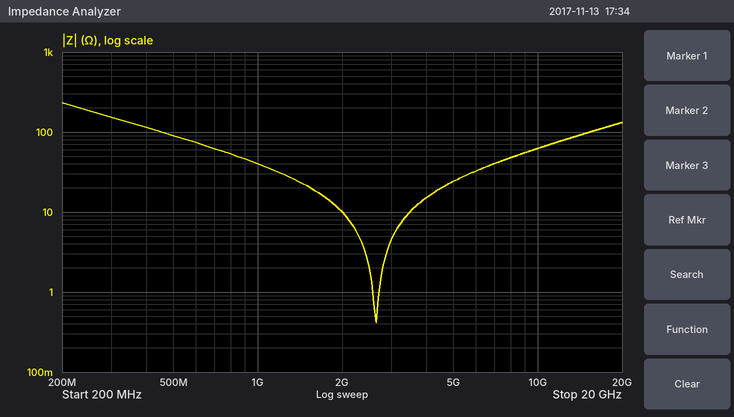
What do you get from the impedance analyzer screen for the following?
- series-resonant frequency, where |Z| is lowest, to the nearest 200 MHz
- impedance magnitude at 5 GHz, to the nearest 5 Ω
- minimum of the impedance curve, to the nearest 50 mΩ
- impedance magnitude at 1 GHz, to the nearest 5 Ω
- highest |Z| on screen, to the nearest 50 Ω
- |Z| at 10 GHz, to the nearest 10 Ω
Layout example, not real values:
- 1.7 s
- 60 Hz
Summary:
- 2.6 GHz
- 25 Ω
- 400 mΩ
- 40 Ω
- 250 Ω
- 60 Ω
